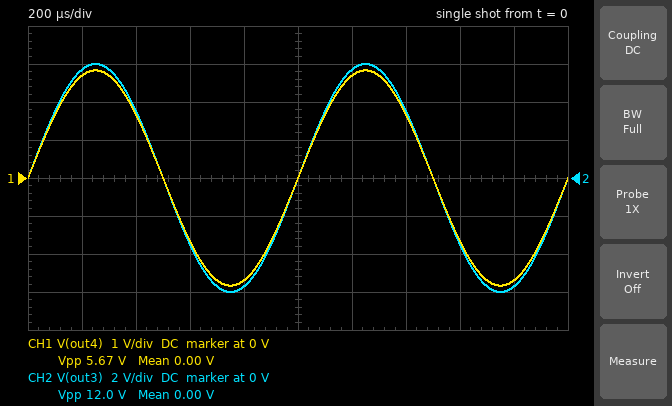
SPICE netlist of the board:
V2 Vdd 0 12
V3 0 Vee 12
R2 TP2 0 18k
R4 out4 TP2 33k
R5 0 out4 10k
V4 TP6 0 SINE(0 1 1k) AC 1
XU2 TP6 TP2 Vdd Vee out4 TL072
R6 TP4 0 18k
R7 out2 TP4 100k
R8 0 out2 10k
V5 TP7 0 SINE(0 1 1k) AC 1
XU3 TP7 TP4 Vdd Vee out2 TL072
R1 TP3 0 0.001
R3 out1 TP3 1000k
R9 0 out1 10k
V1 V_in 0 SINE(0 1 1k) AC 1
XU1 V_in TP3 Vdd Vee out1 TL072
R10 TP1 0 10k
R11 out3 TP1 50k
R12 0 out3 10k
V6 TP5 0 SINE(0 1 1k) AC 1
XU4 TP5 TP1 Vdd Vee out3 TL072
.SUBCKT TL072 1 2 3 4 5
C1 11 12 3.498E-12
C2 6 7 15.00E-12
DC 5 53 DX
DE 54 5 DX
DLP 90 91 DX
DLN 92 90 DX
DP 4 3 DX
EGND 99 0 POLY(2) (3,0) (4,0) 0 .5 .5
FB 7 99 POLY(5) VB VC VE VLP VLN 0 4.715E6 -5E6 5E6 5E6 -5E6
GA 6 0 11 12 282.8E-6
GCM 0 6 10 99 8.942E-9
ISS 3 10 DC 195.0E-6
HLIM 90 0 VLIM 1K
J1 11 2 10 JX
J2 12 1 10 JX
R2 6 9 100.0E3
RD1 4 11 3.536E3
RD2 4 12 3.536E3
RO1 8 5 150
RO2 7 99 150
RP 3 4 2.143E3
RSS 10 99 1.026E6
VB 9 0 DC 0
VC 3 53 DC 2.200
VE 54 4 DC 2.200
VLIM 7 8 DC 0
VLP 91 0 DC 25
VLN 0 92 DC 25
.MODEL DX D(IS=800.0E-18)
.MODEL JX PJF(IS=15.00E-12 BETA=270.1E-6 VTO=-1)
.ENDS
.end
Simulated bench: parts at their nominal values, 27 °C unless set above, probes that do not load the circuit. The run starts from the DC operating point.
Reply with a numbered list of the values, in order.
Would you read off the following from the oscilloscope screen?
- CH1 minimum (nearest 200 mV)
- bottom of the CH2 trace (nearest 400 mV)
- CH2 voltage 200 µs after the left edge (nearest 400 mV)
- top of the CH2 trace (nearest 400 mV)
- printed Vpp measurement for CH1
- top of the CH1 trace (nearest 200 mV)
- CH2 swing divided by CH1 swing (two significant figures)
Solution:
1. -2.8 V
2. -6.0 V
3. 5.6 V
4. 6.0 V
5. 5.67 V
6. 2.8 V
7. 2.1
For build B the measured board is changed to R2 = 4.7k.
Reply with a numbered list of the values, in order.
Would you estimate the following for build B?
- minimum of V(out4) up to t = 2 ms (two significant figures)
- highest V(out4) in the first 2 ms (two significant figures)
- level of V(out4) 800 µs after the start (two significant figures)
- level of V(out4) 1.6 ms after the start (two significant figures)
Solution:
1. -8.0 V
2. 8.0 V
3. -7.6 V
4. -4.7 V
